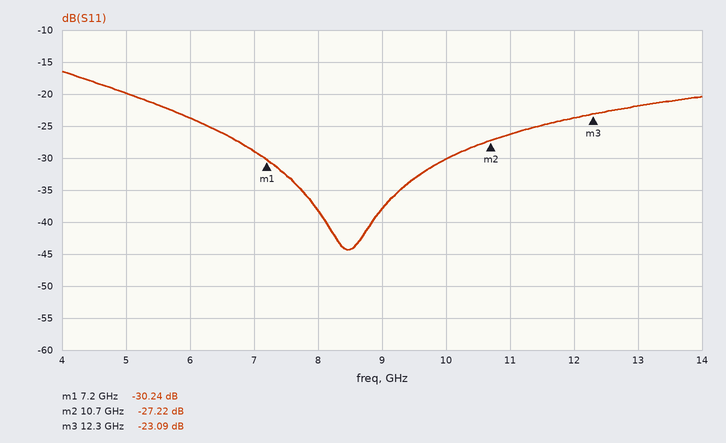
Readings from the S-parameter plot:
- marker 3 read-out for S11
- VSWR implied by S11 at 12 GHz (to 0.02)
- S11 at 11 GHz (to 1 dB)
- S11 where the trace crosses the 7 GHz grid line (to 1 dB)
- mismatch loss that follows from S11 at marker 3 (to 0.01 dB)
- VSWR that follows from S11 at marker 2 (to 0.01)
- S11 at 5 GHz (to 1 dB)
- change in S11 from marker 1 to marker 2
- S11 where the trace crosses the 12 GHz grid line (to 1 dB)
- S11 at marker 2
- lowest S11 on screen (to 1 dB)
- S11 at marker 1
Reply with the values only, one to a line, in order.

-23.09 dB
1.14
-26 dB
-29 dB
0.02 dB
1.09
-20 dB
3.02 dB
-24 dB
-27.22 dB
-44 dB
-30.24 dB
